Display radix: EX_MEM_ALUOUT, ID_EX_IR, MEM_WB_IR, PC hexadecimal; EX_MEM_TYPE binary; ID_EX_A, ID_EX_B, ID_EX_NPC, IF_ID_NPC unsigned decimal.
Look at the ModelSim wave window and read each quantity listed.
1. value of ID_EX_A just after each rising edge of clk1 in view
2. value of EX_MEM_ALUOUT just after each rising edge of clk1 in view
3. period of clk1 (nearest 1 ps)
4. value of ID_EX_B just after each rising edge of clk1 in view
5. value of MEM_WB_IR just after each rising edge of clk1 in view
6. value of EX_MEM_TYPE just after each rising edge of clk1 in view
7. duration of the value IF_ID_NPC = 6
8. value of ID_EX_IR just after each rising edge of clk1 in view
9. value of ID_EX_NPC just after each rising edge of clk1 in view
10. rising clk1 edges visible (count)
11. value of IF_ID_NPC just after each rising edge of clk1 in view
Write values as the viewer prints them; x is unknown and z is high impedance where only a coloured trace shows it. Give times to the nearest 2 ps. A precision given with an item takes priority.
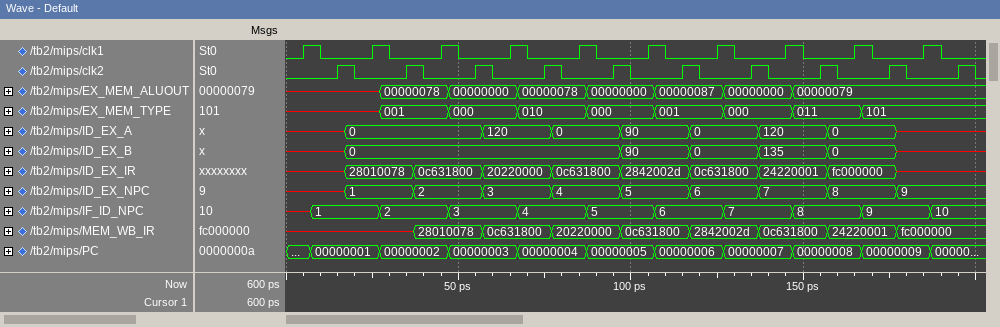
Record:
x, 0, 0, 120, 0, 90, 0, 120, 0, x
x, x, 00000078, 00000000, 00000078, 00000000, 00000087, 00000000, 00000079, 00000079
20 ps
x, 0, 0, 0, 0, 90, 0, 135, 0, x
x, x, 28010078, 0c631800, 20220000, 0c631800, 2842002d, 0c631800, 24220001, fc000000
x, x, 001, 000, 010, 000, 001, 000, 011, 101
20 ps
x, 28010078, 0c631800, 20220000, 0c631800, 2842002d, 0c631800, 24220001, fc000000, x
x, 1, 2, 3, 4, 5, 6, 7, 8, 9
10
x, 1, 2, 3, 4, 5, 6, 7, 8, 9
